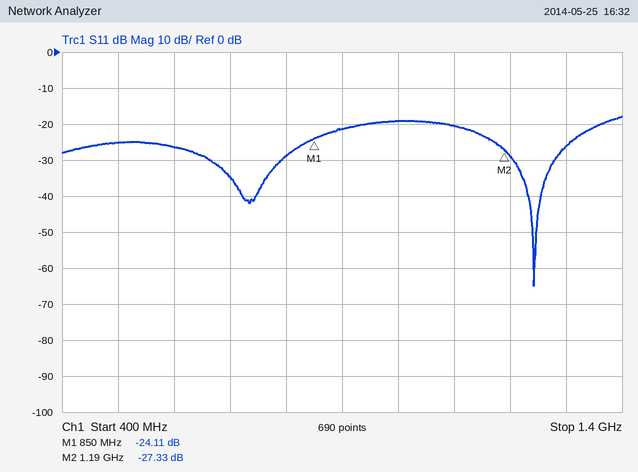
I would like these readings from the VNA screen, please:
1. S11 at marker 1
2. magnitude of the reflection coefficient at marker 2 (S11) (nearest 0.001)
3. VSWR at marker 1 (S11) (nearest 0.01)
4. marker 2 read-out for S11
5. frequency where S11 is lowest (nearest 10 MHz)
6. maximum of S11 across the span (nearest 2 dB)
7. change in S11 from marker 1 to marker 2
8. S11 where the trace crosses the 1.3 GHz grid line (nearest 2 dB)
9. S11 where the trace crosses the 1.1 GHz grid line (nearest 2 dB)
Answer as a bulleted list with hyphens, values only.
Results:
- -24.11 dB
- 0.043
- 1.13
- -27.33 dB
- 1.24 GHz
- -18 dB
- -3.22 dB
- -26 dB
- -20 dB
